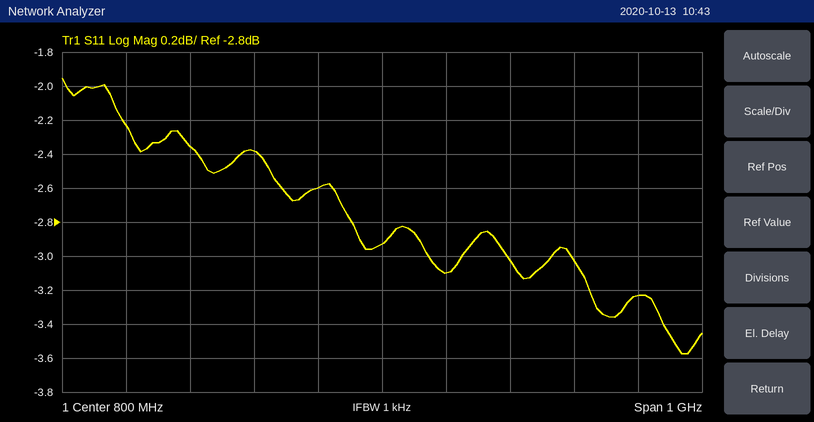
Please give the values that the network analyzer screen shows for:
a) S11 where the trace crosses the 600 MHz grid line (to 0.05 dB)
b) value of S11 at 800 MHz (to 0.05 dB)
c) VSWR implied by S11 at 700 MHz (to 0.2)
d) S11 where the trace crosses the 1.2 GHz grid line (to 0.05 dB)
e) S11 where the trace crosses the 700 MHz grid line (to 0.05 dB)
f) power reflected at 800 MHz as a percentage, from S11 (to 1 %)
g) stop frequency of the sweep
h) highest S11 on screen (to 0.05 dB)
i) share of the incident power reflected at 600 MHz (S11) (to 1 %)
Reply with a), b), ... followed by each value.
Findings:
a) -2.40 dB
b) -2.95 dB
c) 6.8
d) -3.25 dB
e) -2.60 dB
f) 51 %
g) 1.3 GHz
h) -1.95 dB
i) 58 %
